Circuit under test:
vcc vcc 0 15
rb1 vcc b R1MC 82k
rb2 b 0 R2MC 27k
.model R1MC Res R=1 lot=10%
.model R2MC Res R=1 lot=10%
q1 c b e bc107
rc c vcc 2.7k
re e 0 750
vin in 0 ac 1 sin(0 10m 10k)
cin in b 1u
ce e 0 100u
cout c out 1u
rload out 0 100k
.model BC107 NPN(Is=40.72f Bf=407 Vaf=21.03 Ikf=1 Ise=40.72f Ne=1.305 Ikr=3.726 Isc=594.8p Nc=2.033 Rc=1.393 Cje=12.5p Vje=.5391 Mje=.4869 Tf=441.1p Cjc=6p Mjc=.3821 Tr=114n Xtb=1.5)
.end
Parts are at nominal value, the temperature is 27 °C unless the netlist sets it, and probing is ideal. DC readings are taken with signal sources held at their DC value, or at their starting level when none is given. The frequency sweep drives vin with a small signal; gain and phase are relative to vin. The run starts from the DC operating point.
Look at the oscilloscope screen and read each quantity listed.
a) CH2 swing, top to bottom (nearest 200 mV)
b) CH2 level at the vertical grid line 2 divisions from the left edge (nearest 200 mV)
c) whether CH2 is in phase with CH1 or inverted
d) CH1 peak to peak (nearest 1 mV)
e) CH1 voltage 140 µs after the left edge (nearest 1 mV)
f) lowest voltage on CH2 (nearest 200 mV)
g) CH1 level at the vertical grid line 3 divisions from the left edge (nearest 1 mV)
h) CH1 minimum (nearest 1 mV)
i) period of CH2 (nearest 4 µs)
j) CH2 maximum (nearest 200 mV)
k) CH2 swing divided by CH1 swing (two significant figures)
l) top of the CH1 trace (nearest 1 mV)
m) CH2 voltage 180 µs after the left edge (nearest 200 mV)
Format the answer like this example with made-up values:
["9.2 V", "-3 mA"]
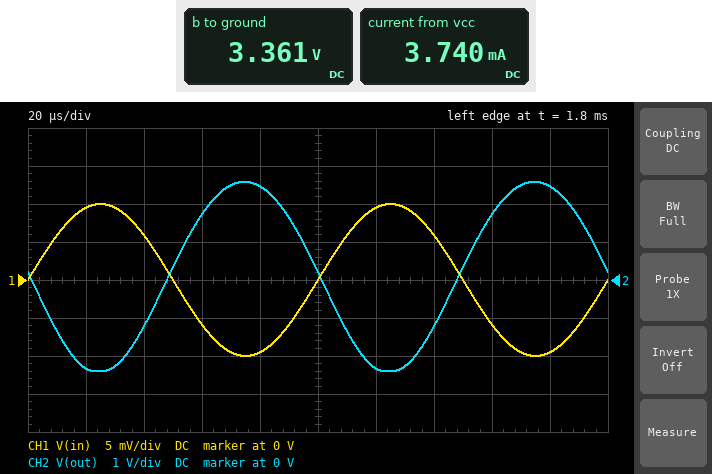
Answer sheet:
["5.0 V", "-1.2 V", "inverted", "20 mV", "6 mV", "-2.4 V", "-6 mV", "-10 mV", "100 µs", "2.6 V", "250", "10 mV", "2.4 V"]
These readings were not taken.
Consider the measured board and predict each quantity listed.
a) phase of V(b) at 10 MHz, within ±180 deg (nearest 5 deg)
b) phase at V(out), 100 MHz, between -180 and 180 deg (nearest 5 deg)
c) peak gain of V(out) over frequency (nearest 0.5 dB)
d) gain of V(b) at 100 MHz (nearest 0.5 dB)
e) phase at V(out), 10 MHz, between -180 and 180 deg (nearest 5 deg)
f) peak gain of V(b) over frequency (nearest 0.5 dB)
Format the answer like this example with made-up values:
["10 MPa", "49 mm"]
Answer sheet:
["0 deg", "100 deg", "48.0 dB", "0 dB", "155 deg", "0 dB"]
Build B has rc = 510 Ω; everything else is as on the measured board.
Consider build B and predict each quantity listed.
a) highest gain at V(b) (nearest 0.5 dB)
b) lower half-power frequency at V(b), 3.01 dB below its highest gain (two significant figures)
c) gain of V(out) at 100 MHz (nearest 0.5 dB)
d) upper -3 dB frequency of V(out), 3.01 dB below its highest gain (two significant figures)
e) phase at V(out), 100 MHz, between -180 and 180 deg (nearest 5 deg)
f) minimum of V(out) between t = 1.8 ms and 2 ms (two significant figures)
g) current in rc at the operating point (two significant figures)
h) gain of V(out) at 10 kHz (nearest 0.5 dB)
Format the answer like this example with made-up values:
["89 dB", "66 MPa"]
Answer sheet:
["0 dB", "20 Hz", "35.0 dB", "150 MHz", "145 deg", "-730 mV", "3.7 mA", "36.5 dB"]
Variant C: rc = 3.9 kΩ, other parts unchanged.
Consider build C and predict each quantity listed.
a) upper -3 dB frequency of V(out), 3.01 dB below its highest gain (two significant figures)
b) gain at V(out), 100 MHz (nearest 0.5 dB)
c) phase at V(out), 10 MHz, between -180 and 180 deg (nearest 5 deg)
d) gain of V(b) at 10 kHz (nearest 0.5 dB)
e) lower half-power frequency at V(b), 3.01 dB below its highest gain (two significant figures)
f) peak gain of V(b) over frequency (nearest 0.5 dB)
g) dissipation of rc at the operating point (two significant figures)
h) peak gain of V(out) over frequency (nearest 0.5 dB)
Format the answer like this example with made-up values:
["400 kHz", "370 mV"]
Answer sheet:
["4.3 MHz", "13.5 dB", "110 deg", "-2.0 dB", "7.7 kHz", "0 dB", "40 mW", "40.5 dB"]
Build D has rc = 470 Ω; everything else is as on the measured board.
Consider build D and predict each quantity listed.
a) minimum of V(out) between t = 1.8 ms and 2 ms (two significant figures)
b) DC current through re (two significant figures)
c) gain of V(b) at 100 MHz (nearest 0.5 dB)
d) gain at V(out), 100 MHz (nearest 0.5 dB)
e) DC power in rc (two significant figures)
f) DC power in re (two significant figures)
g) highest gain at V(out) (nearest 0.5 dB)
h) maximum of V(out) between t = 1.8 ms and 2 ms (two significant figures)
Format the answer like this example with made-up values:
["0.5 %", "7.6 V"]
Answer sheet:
["-680 mV", "3.7 mA", "0 dB", "34.5 dB", "6.5 mW", "10 mW", "36.0 dB", "570 mV"]
